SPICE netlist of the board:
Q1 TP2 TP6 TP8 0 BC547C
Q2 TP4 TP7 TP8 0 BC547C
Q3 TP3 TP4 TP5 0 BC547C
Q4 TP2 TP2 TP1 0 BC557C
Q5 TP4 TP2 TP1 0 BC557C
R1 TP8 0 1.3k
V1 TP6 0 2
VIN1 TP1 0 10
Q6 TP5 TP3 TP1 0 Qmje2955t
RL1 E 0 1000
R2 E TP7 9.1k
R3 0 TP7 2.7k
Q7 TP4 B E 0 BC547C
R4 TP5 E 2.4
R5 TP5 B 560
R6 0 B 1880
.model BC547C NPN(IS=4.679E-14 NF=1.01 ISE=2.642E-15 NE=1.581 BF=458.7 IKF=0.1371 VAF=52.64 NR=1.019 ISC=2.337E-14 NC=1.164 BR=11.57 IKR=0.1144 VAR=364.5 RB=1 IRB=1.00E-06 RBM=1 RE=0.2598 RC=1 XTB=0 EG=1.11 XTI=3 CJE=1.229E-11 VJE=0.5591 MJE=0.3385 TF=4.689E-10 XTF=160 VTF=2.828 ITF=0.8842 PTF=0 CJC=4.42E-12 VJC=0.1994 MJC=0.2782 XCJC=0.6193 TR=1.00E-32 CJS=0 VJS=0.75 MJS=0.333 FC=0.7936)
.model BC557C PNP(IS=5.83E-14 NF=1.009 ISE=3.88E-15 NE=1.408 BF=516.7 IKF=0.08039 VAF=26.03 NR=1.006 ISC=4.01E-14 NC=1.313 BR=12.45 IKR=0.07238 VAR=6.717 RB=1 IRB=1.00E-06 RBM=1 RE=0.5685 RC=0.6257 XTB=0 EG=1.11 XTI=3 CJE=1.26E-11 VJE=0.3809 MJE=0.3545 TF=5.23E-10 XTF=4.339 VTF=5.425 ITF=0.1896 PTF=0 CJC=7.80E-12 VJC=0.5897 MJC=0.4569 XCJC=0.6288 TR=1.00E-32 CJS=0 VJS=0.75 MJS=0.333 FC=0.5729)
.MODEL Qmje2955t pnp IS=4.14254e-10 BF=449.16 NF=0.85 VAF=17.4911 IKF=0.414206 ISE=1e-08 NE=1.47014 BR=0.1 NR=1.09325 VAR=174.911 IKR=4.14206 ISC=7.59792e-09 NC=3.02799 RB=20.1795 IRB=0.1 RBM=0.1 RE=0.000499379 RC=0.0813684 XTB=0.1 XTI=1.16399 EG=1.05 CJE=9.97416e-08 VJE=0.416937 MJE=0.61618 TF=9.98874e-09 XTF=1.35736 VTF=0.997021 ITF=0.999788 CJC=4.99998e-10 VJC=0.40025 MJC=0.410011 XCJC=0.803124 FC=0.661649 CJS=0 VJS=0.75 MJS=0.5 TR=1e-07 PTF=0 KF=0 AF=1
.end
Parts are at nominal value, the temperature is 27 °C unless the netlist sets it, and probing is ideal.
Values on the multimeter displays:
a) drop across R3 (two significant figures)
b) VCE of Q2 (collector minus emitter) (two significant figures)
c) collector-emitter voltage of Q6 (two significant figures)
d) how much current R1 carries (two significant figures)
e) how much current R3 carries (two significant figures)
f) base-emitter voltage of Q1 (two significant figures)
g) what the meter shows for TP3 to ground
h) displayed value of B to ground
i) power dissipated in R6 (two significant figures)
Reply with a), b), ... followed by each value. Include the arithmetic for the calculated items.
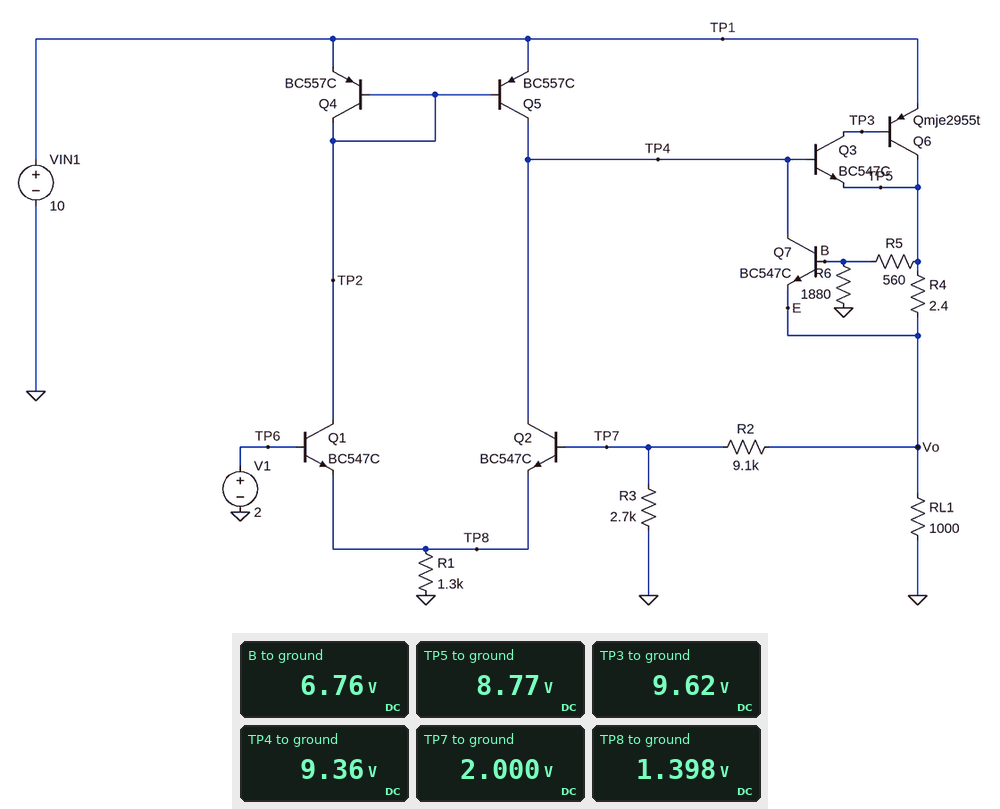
a) 2 V = 2.0 V
b) 9.36 V - 1.398 V = 8.0 V
c) 8.77 V - 10 V = -1.2 V
d) (1.398 V) / 1.3 kΩ = 1.1 mA
e) (2 V) / 2.7 kΩ = 740 µA
f) 2 V - 1.398 V = 600 mV
g) 9.62 V
h) 6.76 V
i) (6.76 V)^2 / 1.88 kΩ = 24 mW
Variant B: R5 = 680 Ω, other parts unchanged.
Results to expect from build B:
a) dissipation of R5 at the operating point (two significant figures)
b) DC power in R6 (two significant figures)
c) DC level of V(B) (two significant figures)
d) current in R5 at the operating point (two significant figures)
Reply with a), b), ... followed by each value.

a) 8.0 mW
b) 22 mW
c) 6.4 V
d) 3.4 mA
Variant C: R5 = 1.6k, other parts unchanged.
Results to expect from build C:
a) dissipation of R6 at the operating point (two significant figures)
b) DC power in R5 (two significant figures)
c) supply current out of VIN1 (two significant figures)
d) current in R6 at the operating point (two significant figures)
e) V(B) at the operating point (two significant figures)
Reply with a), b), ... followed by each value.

a) 12 mW
b) 10 mW
c) 13 mA
d) 2.5 mA
e) 4.7 V
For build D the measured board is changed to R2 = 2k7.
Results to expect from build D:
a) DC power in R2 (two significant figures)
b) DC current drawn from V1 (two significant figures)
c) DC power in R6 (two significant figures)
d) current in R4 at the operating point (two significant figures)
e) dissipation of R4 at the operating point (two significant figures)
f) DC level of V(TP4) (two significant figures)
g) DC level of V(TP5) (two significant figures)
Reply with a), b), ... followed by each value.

a) 1.5 mW
b) 950 nA
c) 5.1 mW
d) 4.8 mA
e) 54 µW
f) 4.6 V
g) 4.0 V
